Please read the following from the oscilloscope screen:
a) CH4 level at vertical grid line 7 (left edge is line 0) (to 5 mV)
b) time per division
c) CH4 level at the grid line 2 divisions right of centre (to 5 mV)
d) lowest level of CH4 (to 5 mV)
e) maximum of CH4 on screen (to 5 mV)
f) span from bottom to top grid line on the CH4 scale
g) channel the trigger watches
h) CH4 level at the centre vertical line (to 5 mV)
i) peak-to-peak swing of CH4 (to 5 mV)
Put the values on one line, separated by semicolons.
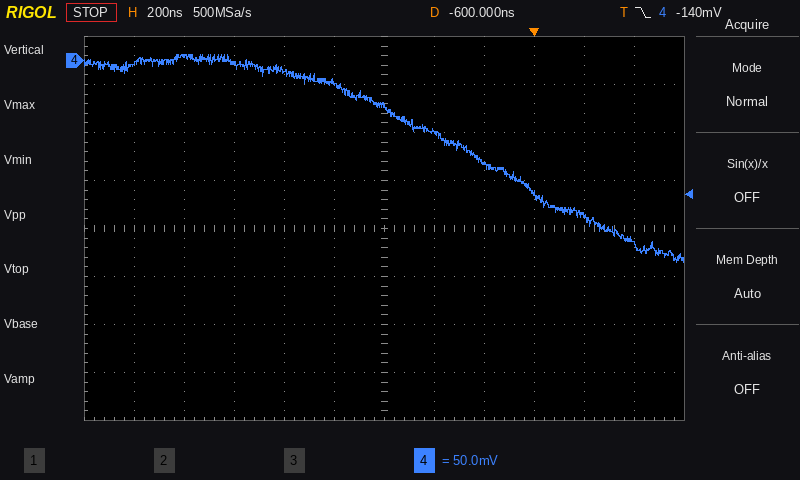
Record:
-75 mV; 200 ns; -110 mV; -210 mV; 5 mV; 400 mV; CH4; -50 mV; 215 mV
